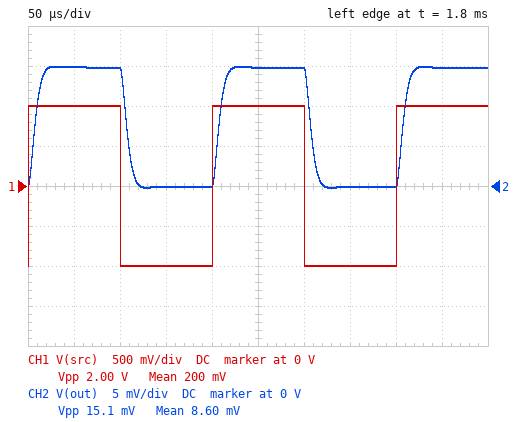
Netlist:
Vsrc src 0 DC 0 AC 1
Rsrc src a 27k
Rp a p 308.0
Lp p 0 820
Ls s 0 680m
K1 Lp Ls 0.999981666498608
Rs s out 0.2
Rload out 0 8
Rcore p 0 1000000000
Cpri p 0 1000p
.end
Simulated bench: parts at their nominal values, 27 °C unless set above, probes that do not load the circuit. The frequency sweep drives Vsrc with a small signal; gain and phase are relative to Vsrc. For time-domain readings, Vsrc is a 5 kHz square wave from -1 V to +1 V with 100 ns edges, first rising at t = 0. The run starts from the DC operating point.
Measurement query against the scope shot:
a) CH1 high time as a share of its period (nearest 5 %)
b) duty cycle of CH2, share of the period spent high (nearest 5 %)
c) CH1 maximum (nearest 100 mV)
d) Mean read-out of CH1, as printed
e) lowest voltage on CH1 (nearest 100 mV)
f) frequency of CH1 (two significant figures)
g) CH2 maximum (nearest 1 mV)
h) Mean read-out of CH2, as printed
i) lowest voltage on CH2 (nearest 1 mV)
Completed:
50 %
50 %
1.0 V
200 mV
-1.0 V
5.0 kHz
15 mV
8.60 mV
0 V
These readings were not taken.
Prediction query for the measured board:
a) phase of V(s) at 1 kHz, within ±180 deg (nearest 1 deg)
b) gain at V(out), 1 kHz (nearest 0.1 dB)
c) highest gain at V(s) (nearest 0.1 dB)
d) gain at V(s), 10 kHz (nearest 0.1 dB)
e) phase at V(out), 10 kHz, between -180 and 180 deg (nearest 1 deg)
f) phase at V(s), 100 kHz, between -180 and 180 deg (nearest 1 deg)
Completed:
-3 deg
-42.5 dB
-42.3 dB
-42.7 dB
-29 deg
-147 deg
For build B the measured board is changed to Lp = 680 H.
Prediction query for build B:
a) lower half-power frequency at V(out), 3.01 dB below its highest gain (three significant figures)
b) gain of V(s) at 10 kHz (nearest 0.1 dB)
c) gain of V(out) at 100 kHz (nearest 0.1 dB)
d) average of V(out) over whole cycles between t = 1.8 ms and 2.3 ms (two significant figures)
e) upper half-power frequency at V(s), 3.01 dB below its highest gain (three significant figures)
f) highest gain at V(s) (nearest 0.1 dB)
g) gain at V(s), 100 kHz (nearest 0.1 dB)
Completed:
1.48 Hz
-42.9 dB
-60.9 dB
7.0 mV
31.6 kHz
-42.7 dB
-60.7 dB
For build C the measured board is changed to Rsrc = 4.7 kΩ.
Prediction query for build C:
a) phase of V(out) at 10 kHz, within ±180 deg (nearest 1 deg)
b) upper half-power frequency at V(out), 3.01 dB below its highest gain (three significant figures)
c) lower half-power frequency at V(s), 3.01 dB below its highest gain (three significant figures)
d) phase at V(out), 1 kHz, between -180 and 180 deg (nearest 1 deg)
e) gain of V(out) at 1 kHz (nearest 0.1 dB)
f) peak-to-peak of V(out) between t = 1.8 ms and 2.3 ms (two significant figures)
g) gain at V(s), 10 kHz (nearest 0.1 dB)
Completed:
-19 deg
41.0 kHz
645 mHz
-2 deg
-34.6 dB
38 mV
-34.5 dB
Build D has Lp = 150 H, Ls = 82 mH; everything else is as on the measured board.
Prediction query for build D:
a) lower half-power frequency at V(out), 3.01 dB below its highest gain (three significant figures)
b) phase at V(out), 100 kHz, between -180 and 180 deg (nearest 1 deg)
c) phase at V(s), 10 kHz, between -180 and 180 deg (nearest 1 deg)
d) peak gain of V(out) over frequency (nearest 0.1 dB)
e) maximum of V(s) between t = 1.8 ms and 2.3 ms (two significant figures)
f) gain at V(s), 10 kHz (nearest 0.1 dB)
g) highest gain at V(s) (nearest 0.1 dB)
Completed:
10.3 Hz
-94 deg
-32 deg
-41.8 dB
16 mV
-42.9 dB
-41.6 dB
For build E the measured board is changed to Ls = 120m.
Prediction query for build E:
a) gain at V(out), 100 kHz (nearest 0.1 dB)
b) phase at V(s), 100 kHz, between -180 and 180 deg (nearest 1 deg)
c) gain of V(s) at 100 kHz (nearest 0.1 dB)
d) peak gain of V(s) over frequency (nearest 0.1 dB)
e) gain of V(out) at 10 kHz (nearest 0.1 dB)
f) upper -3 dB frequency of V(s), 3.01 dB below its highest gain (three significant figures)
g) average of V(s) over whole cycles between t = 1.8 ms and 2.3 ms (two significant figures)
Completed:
-63.7 dB
-104 deg
-63.5 dB
-41.8 dB
-45.6 dB
8.75 kHz
7.8 mV
